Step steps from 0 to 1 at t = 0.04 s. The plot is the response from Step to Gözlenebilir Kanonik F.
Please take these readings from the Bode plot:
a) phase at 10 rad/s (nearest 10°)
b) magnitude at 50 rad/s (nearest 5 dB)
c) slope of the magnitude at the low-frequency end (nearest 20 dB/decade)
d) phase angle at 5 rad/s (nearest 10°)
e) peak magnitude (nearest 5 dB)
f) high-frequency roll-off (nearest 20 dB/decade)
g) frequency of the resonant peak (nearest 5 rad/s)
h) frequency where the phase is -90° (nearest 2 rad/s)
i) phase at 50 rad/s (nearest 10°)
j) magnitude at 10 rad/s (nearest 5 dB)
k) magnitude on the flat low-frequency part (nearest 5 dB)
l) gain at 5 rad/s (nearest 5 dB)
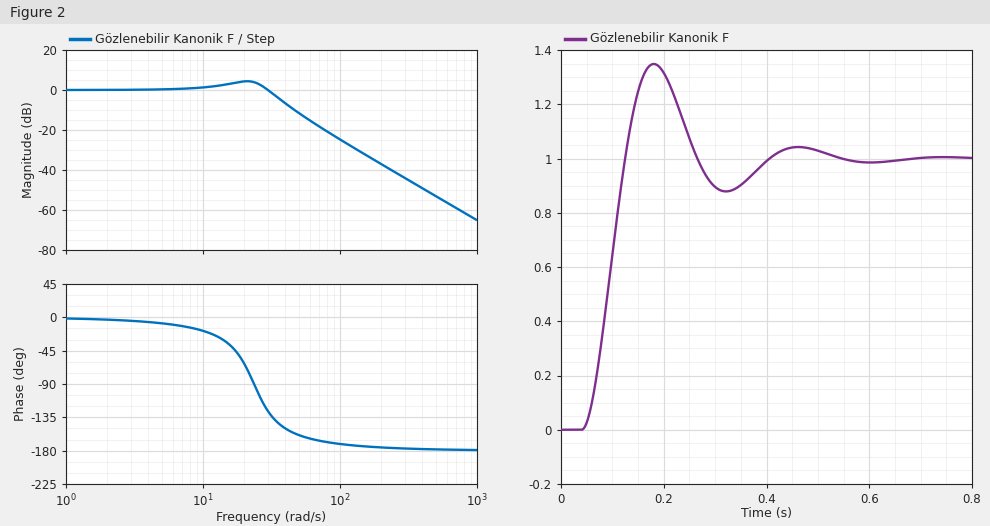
-20°
-10 dB
0 dB/decade
-10°
5 dB
-40 dB/decade
20 rad/s
24 rad/s
-160°
0 dB
0 dB
0 dB
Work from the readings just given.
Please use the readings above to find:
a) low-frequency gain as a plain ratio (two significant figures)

1.0
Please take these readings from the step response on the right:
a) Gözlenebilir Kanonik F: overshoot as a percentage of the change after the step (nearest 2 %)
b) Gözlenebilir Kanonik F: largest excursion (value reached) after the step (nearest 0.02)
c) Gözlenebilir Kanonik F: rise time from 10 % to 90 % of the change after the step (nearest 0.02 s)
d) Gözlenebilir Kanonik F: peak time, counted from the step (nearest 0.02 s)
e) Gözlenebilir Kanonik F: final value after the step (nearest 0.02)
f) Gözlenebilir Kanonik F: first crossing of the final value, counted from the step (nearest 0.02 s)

34 %
1.34
0.06 s
0.14 s
1.00
0.08 s
